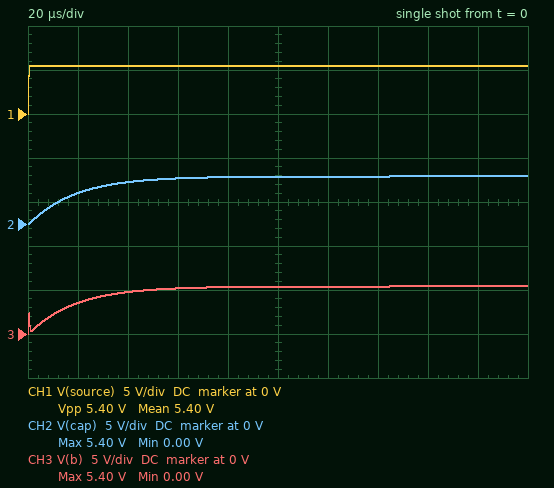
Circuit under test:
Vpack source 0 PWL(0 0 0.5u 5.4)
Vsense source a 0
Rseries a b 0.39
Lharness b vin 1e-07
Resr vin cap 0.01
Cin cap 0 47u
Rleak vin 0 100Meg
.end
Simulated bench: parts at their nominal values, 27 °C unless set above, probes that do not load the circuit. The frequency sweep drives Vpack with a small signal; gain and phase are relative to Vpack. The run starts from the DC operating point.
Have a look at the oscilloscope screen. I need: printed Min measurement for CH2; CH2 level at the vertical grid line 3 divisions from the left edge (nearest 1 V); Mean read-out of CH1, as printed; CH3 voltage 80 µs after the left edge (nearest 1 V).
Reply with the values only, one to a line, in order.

0.00 V
5 V
5.40 V
5 V
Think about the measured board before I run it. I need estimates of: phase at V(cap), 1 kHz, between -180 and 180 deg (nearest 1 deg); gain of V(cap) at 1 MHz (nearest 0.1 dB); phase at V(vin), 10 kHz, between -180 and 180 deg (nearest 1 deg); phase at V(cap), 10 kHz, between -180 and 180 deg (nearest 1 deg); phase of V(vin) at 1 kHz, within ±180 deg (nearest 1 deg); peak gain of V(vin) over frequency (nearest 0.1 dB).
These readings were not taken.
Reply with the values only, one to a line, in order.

-7 deg
-46.8 dB
-49 deg
-50 deg
-7 deg
0 dB
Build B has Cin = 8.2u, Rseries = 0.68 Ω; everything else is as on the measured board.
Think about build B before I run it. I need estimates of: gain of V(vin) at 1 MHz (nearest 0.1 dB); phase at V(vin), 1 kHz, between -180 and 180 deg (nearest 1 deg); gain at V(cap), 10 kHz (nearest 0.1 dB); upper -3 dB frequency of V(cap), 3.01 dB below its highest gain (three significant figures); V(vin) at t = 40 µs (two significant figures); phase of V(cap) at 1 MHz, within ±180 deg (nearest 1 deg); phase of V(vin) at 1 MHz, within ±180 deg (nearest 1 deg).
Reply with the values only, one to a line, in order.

-32.5 dB
-2 deg
-0.5 dB
28.9 kHz
5.4 V
-131 deg
-104 deg
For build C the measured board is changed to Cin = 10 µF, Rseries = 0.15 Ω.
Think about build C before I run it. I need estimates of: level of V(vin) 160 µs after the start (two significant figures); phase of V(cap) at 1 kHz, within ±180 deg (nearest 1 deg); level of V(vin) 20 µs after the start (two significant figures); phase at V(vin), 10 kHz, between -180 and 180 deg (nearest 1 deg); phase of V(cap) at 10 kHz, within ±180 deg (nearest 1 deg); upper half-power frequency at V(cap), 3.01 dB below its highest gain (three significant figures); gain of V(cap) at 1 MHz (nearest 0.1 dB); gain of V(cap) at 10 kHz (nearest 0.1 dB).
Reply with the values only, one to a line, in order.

5.4 V
-1 deg
5.4 V
-5 deg
-6 deg
139 kHz
-32.0 dB
0 dB
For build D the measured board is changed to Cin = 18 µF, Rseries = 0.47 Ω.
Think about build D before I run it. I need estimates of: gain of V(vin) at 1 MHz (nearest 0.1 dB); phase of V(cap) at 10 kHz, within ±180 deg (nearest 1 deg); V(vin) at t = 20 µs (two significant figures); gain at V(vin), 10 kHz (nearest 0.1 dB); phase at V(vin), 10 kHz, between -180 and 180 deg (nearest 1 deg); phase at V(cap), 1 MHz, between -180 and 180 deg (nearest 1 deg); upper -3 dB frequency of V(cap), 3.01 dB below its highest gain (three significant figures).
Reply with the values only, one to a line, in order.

-35.4 dB
-29 deg
4.9 V
-1.1 dB
-28 deg
-142 deg
18.9 kHz
